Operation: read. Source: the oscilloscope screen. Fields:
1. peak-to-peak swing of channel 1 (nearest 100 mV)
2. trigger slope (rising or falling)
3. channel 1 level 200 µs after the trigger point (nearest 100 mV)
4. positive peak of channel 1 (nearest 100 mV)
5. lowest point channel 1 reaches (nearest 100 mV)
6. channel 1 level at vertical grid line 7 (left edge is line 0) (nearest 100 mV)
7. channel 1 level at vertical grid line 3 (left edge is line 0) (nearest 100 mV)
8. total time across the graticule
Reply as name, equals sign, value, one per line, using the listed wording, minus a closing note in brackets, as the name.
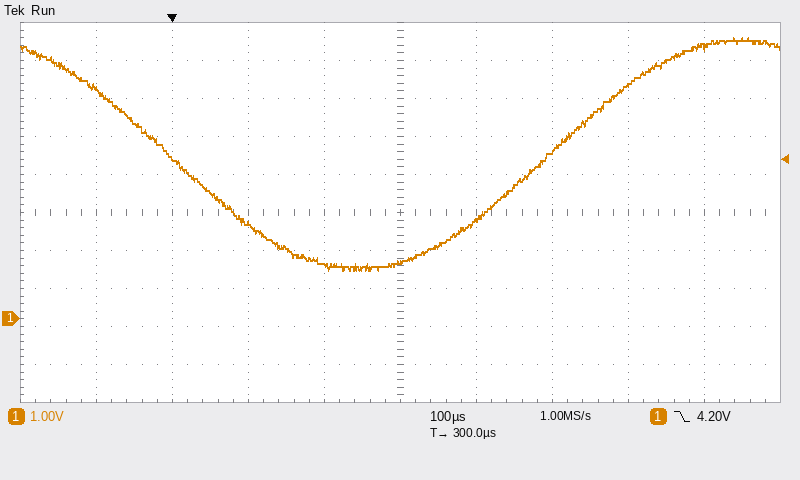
peak-to-peak swing of channel 1 = 6.1 V
trigger slope = falling
channel 1 level 200 µs after the trigger point = 1.4 V
positive peak of channel 1 = 7.4 V
lowest point channel 1 reaches = 1.3 V
channel 1 level at vertical grid line 7 (left edge is line 0) = 4.4 V
channel 1 level at vertical grid line 3 (left edge is line 0) = 2.5 V
total time across the graticule = 1 ms
